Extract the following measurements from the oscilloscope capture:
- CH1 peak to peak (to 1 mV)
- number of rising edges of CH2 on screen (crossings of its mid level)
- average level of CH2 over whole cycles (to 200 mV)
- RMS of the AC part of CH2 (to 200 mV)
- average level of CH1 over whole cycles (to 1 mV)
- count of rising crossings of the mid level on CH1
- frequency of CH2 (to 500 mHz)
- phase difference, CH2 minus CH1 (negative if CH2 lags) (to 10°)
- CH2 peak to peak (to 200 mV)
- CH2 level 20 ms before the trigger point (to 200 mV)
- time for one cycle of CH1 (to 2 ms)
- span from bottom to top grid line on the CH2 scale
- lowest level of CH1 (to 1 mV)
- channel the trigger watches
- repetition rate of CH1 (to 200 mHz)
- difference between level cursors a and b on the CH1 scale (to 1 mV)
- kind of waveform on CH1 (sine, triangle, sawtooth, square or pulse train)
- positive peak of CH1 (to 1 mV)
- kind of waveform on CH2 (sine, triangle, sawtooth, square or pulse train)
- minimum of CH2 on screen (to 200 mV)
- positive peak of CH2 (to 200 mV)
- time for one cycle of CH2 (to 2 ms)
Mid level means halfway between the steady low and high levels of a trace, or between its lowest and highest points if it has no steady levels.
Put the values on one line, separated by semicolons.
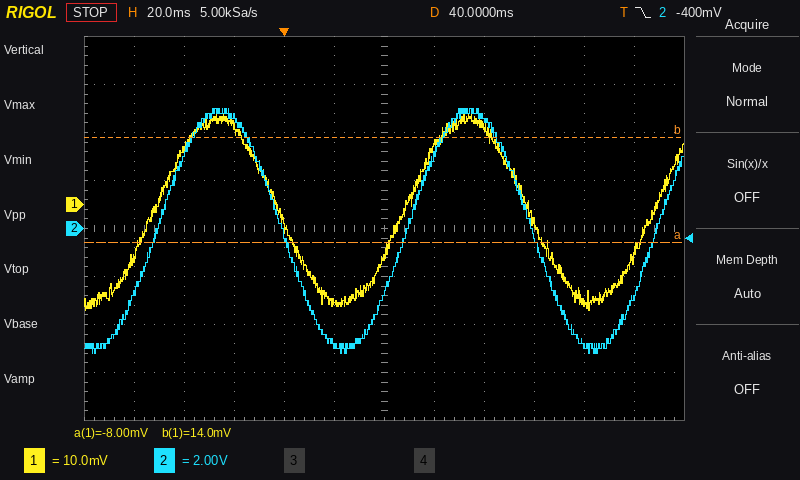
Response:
41 mV; 3; 0.0 V; 3.6 V; -1 mV; 3; 10.0 Hz; 0°; 10.2 V; 4.6 V; 100 ms; 16 V; -22 mV; CH2; 10.0 Hz; 22 mV; sine; 19 mV; sine; -5.2 V; 5.0 V; 100 ms
